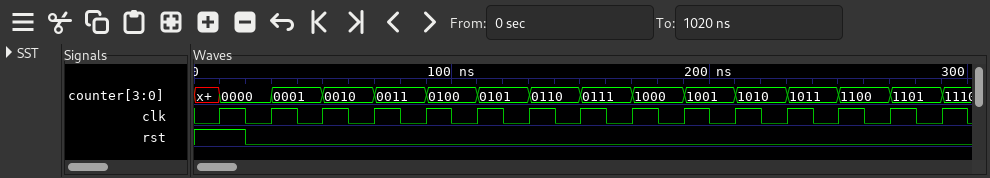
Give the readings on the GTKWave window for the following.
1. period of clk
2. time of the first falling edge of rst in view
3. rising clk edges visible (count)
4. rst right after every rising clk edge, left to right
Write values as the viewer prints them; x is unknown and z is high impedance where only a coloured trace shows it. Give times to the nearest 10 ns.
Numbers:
20 ns
20 ns
15
1 0 0 0 0 0 0 0 0 0 0 0 0 0 0
